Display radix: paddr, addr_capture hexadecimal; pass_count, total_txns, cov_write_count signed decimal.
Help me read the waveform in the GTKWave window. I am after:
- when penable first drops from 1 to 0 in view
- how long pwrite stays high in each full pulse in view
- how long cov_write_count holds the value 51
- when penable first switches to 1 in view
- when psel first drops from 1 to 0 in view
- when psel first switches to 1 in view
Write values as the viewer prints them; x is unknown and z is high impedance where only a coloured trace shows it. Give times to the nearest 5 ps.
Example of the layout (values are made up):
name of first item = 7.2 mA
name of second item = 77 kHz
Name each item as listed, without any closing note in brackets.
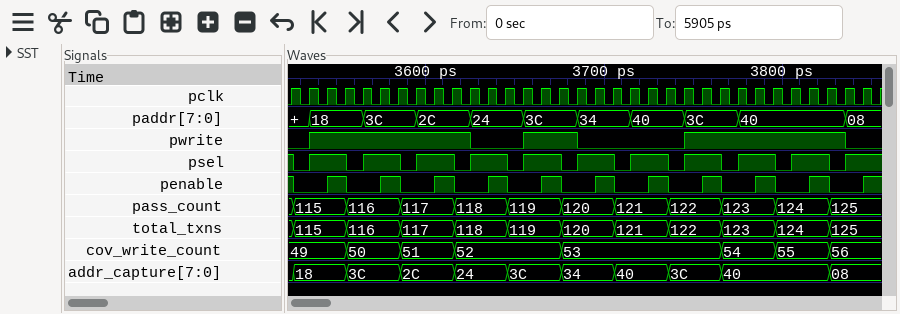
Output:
when penable first drops from 1 to 0 in view = 3525 ps
how long pwrite stays high in each full pulse in view = 90 ps, 30 ps, 90 ps
how long cov_write_count holds the value 51 = 30 ps
when penable first switches to 1 in view = 3545 ps
when psel first drops from 1 to 0 in view = 3525 ps
when psel first switches to 1 in view = 3535 ps
